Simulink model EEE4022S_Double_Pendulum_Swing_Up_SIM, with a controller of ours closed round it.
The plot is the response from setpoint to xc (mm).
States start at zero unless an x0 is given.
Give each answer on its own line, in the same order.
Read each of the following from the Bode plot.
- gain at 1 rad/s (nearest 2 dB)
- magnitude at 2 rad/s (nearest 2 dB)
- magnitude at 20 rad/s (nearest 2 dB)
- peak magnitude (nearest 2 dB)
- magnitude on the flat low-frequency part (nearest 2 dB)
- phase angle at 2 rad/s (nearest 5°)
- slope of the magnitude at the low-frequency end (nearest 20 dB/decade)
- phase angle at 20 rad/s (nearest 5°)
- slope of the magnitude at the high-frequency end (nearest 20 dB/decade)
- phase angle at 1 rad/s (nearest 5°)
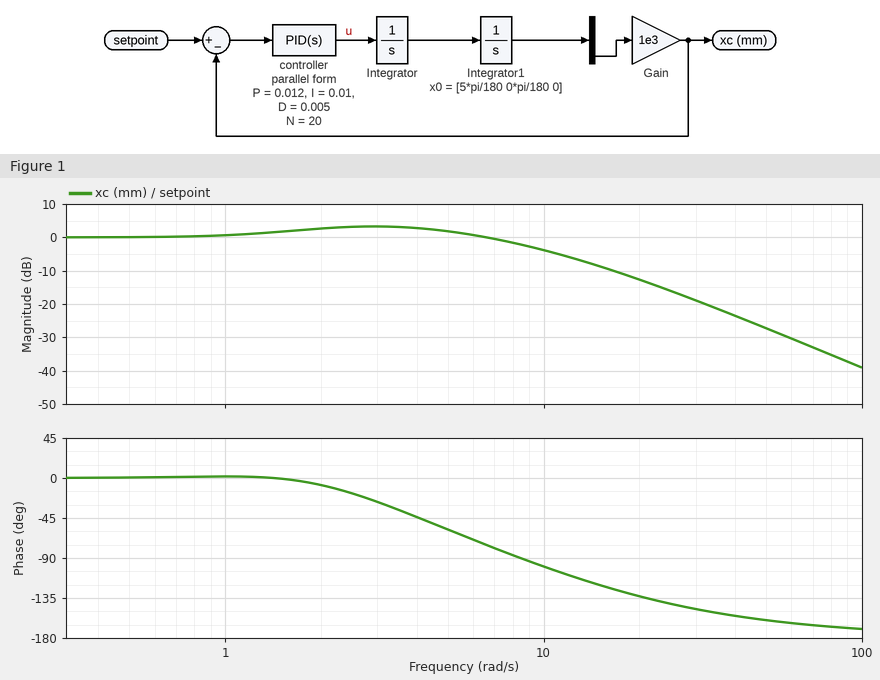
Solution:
0 dB
2 dB
-12 dB
4 dB
0 dB
-10°
0 dB/decade
-135°
-40 dB/decade
0°
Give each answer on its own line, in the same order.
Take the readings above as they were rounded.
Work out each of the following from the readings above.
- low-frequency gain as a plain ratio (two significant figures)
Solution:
1.0
